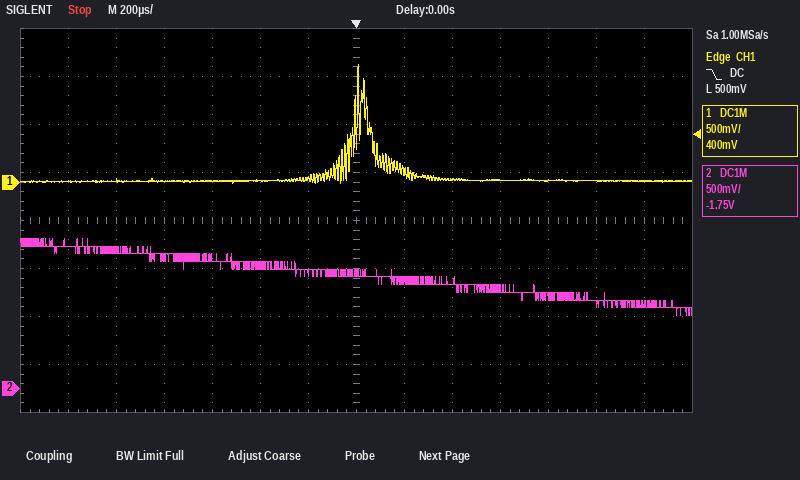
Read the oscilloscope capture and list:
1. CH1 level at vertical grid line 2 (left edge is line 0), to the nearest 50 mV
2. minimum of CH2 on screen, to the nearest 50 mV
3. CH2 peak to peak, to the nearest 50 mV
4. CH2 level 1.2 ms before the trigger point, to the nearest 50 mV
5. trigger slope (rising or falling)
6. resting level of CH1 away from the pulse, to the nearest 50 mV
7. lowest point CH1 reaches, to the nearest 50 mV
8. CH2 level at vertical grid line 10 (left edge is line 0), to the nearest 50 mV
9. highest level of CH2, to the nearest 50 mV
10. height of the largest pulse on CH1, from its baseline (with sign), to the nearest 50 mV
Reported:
0 mV
750 mV
800 mV
1.50 V
falling
0 mV
0 mV
1.05 V
1.55 V
+1.20 V
